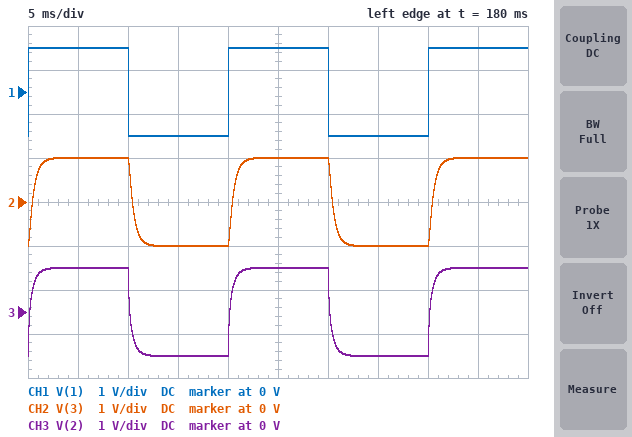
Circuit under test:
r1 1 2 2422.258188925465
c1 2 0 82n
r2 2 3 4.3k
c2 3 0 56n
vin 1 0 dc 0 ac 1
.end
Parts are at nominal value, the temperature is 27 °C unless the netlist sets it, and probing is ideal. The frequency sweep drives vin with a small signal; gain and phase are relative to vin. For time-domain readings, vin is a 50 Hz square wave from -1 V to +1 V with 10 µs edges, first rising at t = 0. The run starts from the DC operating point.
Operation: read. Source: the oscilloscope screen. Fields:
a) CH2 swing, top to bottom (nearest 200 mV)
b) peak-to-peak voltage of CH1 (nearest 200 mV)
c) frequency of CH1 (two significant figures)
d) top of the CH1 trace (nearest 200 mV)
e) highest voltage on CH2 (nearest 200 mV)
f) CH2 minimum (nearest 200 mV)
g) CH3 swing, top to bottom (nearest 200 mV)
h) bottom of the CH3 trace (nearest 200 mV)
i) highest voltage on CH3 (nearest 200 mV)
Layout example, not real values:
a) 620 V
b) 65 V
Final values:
a) 2.0 V
b) 2.0 V
c) 50 Hz
d) 1.0 V
e) 1.0 V
f) -1.0 V
g) 2.0 V
h) -1.0 V
i) 1.0 V
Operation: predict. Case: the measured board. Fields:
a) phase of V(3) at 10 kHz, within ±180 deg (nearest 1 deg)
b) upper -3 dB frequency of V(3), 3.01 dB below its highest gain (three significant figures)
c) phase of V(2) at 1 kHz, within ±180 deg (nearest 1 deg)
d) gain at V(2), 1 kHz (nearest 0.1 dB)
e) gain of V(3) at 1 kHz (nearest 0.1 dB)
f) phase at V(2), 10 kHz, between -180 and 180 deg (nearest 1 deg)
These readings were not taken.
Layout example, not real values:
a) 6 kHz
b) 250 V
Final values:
a) -169 deg
b) 322 Hz
c) -47 deg
d) -6.2 dB
e) -11.4 dB
f) -83 deg
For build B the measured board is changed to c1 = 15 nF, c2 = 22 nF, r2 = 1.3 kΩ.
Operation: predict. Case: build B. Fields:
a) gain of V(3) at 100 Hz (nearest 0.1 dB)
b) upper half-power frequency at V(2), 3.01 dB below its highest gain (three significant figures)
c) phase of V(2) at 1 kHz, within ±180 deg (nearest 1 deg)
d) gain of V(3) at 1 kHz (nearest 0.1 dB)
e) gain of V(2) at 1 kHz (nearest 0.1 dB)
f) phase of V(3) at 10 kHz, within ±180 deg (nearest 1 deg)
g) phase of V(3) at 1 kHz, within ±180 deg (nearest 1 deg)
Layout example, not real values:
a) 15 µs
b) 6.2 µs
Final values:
a) 0 dB
b) 1.56 kHz
c) -28 deg
d) -1.7 dB
e) -1.5 dB
f) -113 deg
g) -38 deg
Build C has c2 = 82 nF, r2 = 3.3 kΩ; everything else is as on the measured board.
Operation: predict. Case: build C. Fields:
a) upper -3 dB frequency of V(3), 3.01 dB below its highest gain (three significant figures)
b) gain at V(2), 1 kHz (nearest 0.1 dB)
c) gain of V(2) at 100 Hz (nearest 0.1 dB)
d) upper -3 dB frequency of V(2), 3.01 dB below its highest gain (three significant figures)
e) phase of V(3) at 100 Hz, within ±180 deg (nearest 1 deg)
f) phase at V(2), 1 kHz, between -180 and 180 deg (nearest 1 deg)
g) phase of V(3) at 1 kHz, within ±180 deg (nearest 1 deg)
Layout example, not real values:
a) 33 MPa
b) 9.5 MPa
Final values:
a) 270 Hz
b) -6.9 dB
c) -0.4 dB
d) 351 Hz
e) -23 deg
f) -45 deg
g) -105 deg
